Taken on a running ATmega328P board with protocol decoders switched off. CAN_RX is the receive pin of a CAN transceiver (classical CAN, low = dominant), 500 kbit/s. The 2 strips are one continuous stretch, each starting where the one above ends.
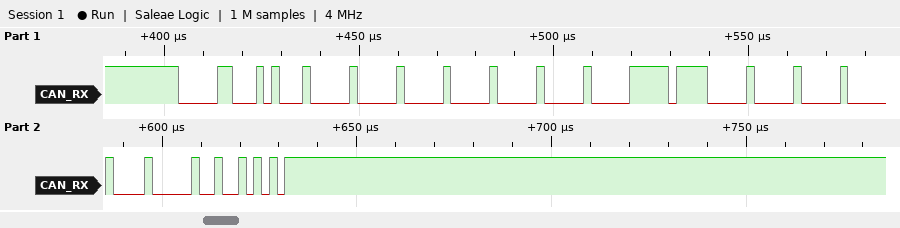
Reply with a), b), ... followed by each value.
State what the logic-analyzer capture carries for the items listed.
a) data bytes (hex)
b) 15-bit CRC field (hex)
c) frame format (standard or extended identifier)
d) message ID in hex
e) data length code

a) 00 00 00 00 FF 00 00 00
b) 0x404A
c) standard
d) 0x045
e) 8
